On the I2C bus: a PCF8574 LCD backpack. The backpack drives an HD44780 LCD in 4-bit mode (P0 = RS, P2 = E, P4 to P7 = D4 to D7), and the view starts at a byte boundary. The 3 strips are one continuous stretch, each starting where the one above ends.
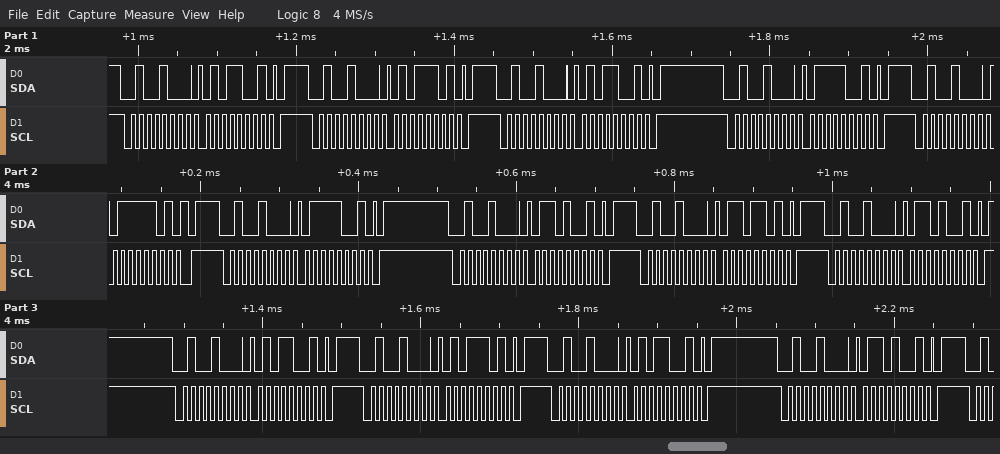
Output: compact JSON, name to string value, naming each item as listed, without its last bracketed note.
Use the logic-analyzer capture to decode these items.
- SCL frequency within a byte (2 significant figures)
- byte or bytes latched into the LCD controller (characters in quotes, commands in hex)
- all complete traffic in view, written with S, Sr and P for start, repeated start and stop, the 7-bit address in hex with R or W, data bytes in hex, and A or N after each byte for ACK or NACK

{"SCL frequency within a byte": "100 kHz", "byte or bytes latched into the LCD controller": "'W' 'e'", "all complete traffic in view, written with S, Sr and P for start, repeated start and stop, the 7-bit address in hex with R or W, data bytes in hex, and A or N after each byte for ACK or NACK": "S 24W A 59 A P S 24W A 5D A P S 24W A 59 A P S 24W A 79 A P S 24W A 7D A P S 24W A 79 A P S 24W A 69 A P S 24W A 6D A P S 24W A 69 A P S 24W A 59 A P S 24W A 5D A P S 24W A 59 A P S 24W A 69 A P"}
